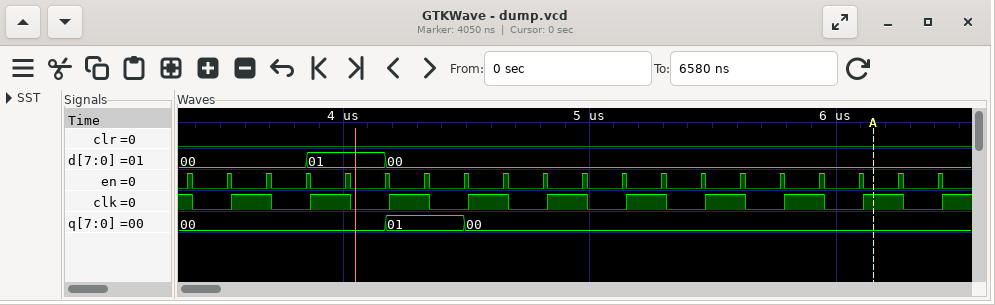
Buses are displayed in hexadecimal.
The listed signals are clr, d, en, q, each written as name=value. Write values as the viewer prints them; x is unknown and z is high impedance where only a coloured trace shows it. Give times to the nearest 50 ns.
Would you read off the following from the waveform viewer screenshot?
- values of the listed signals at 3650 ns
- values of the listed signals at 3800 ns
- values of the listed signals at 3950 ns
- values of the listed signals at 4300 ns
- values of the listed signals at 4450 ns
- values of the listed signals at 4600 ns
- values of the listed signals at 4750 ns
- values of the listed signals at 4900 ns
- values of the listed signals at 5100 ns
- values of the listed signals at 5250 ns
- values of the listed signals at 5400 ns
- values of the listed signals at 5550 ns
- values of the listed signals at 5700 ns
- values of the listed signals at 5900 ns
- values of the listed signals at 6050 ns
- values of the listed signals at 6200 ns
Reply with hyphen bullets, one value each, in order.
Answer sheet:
- clr=0, d=00, en=0, q=00
- clr=0, d=00, en=0, q=00
- clr=0, d=01, en=0, q=00
- clr=0, d=00, en=0, q=01
- clr=0, d=00, en=0, q=01
- clr=0, d=00, en=0, q=00
- clr=0, d=00, en=0, q=00
- clr=0, d=00, en=0, q=00
- clr=0, d=00, en=0, q=00
- clr=0, d=00, en=0, q=00
- clr=0, d=00, en=0, q=00
- clr=0, d=00, en=0, q=00
- clr=0, d=00, en=0, q=00
- clr=0, d=00, en=0, q=00
- clr=0, d=00, en=0, q=00
- clr=0, d=00, en=0, q=00
